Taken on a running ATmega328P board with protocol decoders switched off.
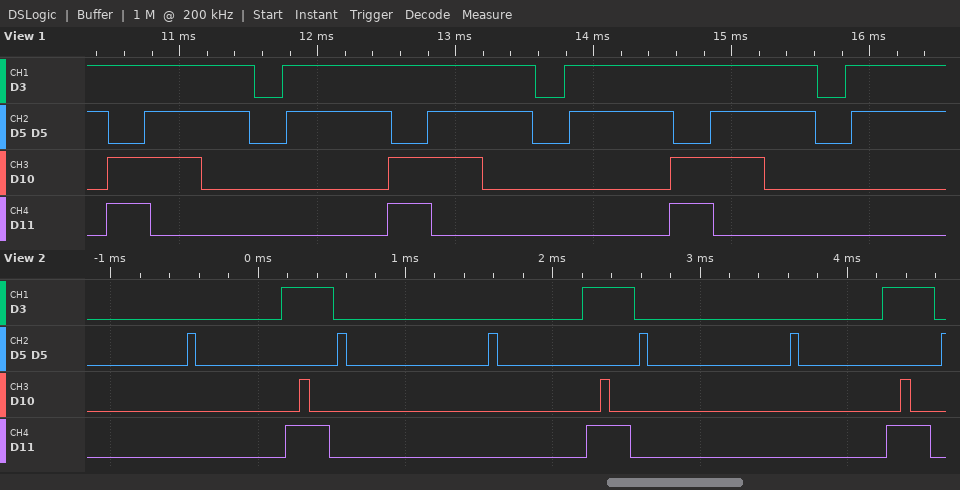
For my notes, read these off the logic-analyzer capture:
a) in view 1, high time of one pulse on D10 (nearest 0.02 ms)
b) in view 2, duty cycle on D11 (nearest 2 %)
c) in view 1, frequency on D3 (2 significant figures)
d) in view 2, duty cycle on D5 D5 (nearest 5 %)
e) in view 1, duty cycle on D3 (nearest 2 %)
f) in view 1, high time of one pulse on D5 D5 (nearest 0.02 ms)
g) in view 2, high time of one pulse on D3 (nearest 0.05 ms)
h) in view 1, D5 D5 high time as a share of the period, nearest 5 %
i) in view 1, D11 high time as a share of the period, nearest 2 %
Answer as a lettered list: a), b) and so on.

a) 0.68 ms
b) 14 %
c) 490 Hz
d) 5 %
e) 90 %
f) 0.76 ms
g) 0.35 ms
h) 75 %
i) 16 %
